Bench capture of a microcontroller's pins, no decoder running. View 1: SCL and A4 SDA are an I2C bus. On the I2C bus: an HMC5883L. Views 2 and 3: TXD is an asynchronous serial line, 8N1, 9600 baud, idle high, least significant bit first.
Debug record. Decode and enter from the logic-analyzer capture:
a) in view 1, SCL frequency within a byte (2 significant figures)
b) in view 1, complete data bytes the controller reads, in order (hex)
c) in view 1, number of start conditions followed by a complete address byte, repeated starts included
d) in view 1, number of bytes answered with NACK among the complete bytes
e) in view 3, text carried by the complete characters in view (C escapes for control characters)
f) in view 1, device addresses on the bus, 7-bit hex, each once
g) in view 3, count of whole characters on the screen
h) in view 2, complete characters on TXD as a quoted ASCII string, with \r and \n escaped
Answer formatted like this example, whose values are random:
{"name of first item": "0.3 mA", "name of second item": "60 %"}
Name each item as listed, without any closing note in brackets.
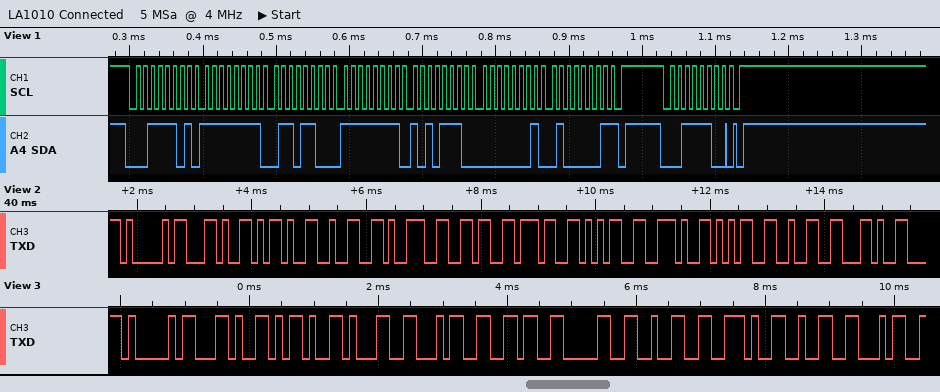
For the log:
{"in view 1, SCL frequency within a byte": "100 kHz", "in view 1, complete data bytes the controller reads, in order": "FF 6C FF AE 01 41", "in view 1, number of start conditions followed by a complete address byte, repeated starts included": "2", "in view 1, number of bytes answered with NACK among the complete bytes": "1", "in view 3, text carried by the complete characters in view": "\"A,-14602.24\"", "in view 1, device addresses on the bus, 7-bit hex, each once": "0x1E", "in view 3, count of whole characters on the screen": "11", "in view 2, complete characters on TXD as a quoted ASCII string, with \\r and \\n escaped": "\"A,-29675.52,\""}
